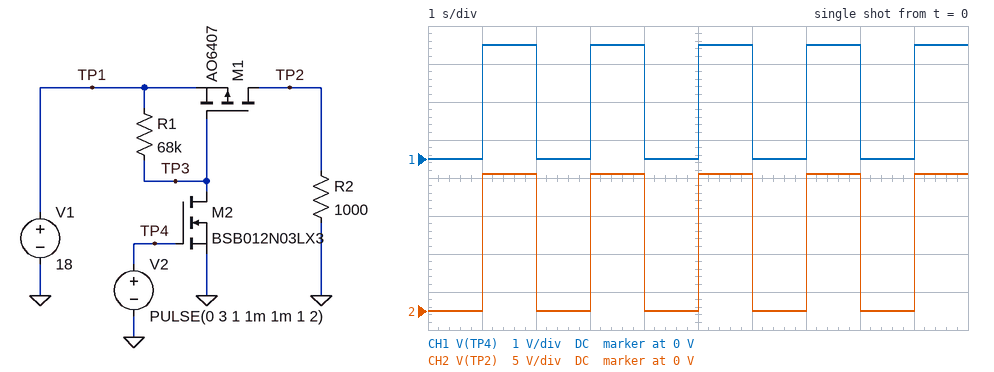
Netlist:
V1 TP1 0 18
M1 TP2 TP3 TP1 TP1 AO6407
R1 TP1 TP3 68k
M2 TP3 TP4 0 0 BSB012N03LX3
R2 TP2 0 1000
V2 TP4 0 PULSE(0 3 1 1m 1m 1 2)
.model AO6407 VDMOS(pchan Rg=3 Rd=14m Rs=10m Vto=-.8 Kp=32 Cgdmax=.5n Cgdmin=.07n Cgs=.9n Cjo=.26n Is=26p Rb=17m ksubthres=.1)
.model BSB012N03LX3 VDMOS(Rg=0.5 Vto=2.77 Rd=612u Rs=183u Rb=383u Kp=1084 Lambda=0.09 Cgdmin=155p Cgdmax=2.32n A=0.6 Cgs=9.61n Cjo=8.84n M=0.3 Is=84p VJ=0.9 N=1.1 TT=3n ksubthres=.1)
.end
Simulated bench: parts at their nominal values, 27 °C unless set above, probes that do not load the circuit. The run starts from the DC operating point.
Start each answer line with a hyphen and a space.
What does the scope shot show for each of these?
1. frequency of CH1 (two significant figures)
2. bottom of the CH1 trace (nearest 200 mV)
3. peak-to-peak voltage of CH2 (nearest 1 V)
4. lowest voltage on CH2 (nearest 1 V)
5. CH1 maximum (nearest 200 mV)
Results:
- 500 mHz
- 0 V
- 18 V
- 0 V
- 3.0 V
